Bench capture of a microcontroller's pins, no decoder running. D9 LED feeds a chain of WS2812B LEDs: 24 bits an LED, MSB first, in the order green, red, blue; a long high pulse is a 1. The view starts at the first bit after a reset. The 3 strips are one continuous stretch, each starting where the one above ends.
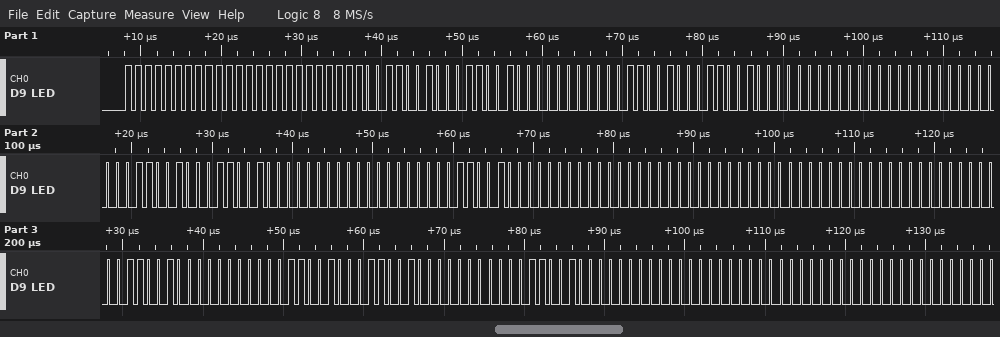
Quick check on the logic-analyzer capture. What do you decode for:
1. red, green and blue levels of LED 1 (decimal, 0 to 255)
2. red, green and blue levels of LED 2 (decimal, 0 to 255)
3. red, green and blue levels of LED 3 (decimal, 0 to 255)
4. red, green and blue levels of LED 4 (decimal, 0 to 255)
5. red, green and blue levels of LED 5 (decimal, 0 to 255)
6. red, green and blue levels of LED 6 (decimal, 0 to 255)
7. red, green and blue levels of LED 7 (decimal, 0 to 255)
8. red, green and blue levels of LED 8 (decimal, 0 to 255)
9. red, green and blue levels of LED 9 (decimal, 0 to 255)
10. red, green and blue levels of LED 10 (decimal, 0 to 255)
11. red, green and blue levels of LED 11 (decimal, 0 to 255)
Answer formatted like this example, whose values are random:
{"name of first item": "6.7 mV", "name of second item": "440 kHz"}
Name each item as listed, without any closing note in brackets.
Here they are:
{"red, green and blue levels of LED 1": "255, 255, 255", "red, green and blue levels of LED 2": "50, 50, 0", "red, green and blue levels of LED 3": "50, 50, 0", "red, green and blue levels of LED 4": "0, 0, 50", "red, green and blue levels of LED 5": "0, 50, 0", "red, green and blue levels of LED 6": "0, 50, 0", "red, green and blue levels of LED 7": "0, 0, 0", "red, green and blue levels of LED 8": "50, 0, 0", "red, green and blue levels of LED 9": "50, 50, 0", "red, green and blue levels of LED 10": "0, 50, 0", "red, green and blue levels of LED 11": "0, 0, 0"}
